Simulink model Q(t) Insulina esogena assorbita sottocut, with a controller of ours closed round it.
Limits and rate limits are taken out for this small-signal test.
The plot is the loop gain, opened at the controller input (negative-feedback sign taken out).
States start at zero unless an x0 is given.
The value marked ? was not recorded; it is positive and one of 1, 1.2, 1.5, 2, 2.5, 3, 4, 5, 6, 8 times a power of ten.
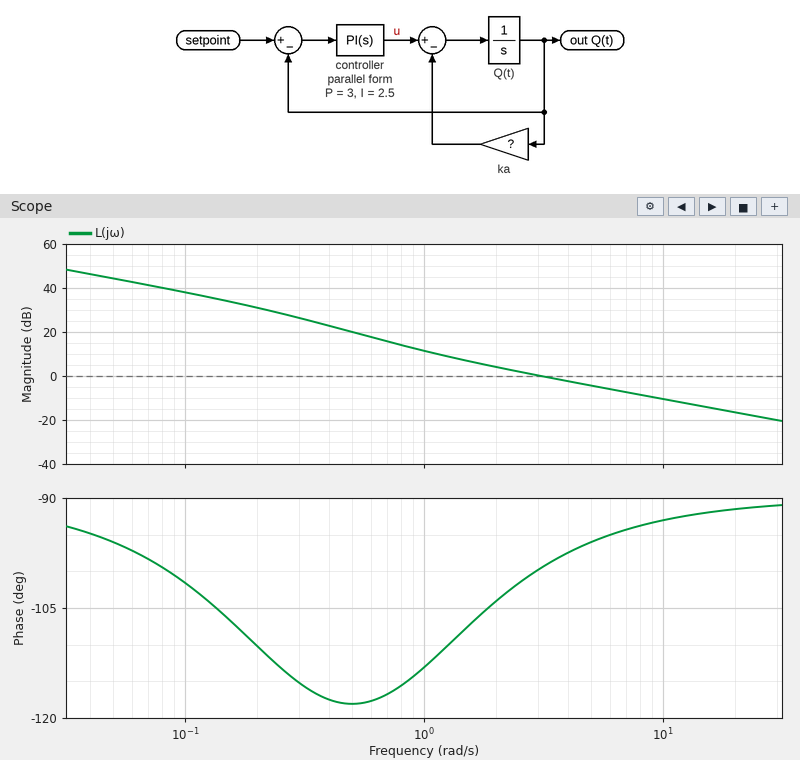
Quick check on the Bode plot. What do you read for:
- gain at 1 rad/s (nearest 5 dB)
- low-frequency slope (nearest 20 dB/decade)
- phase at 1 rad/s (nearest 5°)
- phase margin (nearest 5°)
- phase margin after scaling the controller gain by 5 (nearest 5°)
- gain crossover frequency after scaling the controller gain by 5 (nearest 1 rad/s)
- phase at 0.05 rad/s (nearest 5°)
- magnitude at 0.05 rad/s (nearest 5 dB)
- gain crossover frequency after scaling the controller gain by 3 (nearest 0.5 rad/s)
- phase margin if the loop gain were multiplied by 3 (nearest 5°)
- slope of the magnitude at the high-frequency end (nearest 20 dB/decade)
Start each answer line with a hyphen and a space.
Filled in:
- 10 dB
- -20 dB/decade
- -115°
- 80°
- 90°
- 15 rad/s
- -95°
- 45 dB
- 9.0 rad/s
- 85°
- -20 dB/decade
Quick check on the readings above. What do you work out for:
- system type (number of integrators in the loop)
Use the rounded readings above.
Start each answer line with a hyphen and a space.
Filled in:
- 1
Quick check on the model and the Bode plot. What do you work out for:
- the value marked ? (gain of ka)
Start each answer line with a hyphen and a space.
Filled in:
- 0.3
